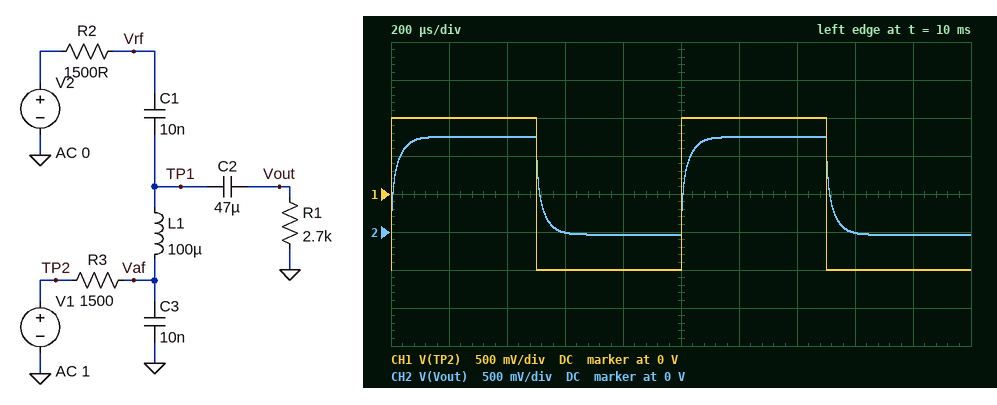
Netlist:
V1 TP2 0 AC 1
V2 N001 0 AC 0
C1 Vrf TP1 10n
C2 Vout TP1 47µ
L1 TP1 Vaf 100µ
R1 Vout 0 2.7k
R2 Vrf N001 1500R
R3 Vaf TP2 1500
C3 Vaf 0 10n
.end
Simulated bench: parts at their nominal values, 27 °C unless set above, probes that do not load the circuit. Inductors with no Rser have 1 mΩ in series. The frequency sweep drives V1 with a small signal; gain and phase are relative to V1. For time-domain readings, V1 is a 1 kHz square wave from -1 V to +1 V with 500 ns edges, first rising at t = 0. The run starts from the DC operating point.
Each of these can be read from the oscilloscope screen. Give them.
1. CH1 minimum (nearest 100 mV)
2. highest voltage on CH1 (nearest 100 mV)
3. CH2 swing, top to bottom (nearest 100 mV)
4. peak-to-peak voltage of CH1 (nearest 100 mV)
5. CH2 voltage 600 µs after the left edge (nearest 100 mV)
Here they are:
-1.0 V
1.0 V
1.3 V
2.0 V
0 V
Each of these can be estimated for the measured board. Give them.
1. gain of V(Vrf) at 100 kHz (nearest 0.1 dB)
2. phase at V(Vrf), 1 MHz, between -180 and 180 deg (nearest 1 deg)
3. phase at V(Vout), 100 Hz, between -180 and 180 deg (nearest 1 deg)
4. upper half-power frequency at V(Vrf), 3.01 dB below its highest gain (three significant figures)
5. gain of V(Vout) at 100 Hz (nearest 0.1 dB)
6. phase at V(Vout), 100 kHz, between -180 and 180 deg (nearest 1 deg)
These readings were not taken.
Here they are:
-19.8 dB
-121 deg
0 deg
42.4 kHz
-3.8 dB
-79 deg
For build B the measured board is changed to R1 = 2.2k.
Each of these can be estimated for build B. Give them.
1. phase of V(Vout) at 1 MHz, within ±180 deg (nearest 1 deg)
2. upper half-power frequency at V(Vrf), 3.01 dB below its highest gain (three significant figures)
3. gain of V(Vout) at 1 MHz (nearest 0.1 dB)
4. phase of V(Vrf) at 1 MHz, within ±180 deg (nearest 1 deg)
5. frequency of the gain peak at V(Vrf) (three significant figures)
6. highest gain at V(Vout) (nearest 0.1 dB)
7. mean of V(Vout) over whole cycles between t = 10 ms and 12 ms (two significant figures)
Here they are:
-124 deg
44.0 kHz
-41.1 dB
-123 deg
13.9 kHz
-4.5 dB
560 mV
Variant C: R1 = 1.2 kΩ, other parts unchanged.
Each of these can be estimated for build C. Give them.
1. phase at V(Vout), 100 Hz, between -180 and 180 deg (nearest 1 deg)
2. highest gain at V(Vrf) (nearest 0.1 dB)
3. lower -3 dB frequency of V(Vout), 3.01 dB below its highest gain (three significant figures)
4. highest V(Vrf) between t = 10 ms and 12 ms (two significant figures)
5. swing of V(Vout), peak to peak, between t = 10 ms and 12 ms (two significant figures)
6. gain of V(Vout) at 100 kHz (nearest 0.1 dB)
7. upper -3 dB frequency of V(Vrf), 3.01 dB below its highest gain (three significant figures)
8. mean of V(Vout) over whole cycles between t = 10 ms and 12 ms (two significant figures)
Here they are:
0 deg
-12.5 dB
1.25 Hz
390 mV
890 mV
-19.9 dB
51.2 kHz
410 mV
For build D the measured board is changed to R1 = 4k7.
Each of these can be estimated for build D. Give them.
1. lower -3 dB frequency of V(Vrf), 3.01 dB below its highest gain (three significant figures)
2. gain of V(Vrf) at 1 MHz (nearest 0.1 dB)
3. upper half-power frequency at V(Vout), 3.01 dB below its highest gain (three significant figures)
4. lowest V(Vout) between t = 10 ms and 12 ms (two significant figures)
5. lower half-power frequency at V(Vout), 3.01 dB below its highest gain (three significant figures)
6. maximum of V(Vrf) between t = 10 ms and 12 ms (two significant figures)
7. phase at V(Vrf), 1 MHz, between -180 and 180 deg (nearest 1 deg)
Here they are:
3.82 kHz
-40.6 dB
6.13 kHz
-31 mV
546 mHz
500 mV
-117 deg
